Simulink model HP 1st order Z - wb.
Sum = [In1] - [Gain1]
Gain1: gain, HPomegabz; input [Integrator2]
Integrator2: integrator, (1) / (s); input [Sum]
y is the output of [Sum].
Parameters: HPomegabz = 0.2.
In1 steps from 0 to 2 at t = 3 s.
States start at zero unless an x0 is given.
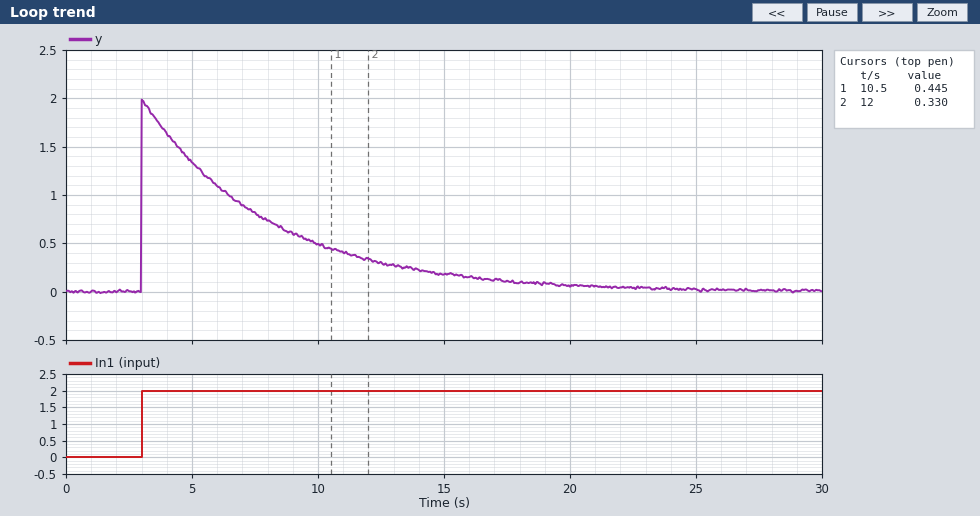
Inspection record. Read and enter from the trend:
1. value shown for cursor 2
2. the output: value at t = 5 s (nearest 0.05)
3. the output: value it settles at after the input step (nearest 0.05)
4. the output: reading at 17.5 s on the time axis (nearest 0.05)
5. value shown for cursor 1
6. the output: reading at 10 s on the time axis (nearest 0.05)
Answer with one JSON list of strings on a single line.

["0.330", "1.35", "0.00", "0.10", "0.445", "0.50"]
